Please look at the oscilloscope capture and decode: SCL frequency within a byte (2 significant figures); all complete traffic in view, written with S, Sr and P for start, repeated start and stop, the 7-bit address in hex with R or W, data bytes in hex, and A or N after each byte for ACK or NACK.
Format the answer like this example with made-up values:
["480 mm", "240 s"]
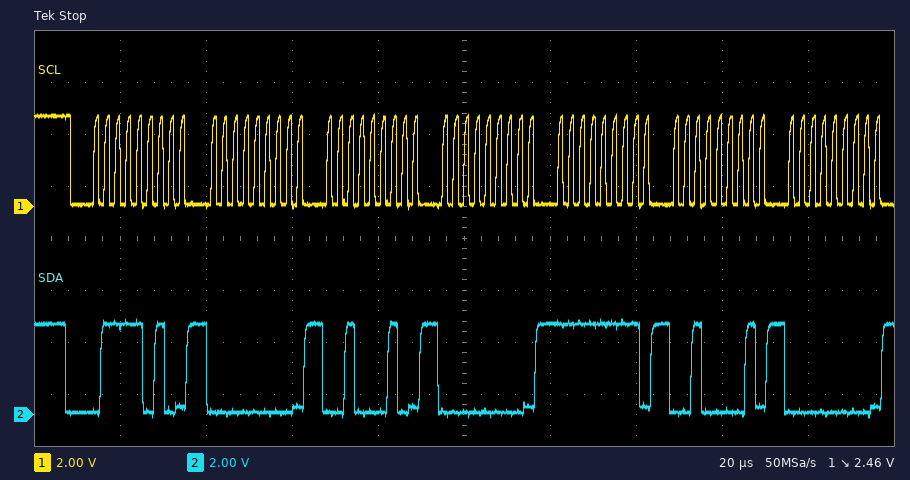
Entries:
["400 kHz", "S 3DW A 00 A 22 A 00 A FF A 21 A 00 A"]
